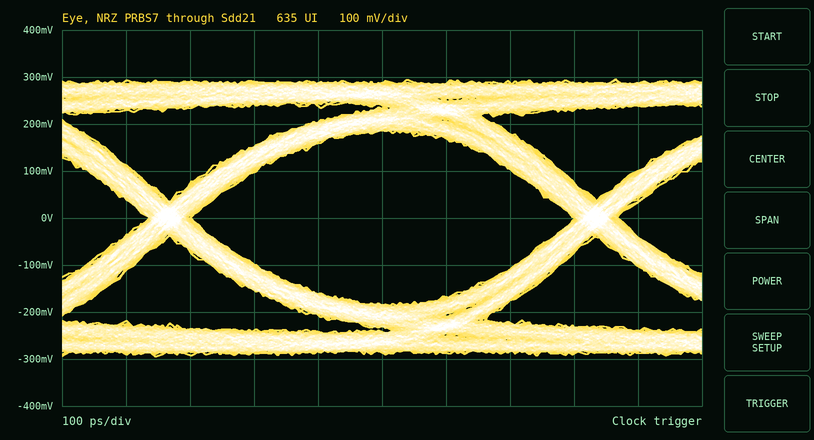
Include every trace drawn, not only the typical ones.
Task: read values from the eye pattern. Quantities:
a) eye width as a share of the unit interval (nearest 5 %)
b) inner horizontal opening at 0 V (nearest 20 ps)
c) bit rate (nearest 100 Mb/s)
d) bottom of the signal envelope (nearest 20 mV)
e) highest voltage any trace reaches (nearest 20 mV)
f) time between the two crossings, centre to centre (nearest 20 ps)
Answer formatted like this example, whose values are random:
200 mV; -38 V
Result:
90 %; 600 ps; 1.5 Gb/s; -300 mV; 300 mV; 660 ps
